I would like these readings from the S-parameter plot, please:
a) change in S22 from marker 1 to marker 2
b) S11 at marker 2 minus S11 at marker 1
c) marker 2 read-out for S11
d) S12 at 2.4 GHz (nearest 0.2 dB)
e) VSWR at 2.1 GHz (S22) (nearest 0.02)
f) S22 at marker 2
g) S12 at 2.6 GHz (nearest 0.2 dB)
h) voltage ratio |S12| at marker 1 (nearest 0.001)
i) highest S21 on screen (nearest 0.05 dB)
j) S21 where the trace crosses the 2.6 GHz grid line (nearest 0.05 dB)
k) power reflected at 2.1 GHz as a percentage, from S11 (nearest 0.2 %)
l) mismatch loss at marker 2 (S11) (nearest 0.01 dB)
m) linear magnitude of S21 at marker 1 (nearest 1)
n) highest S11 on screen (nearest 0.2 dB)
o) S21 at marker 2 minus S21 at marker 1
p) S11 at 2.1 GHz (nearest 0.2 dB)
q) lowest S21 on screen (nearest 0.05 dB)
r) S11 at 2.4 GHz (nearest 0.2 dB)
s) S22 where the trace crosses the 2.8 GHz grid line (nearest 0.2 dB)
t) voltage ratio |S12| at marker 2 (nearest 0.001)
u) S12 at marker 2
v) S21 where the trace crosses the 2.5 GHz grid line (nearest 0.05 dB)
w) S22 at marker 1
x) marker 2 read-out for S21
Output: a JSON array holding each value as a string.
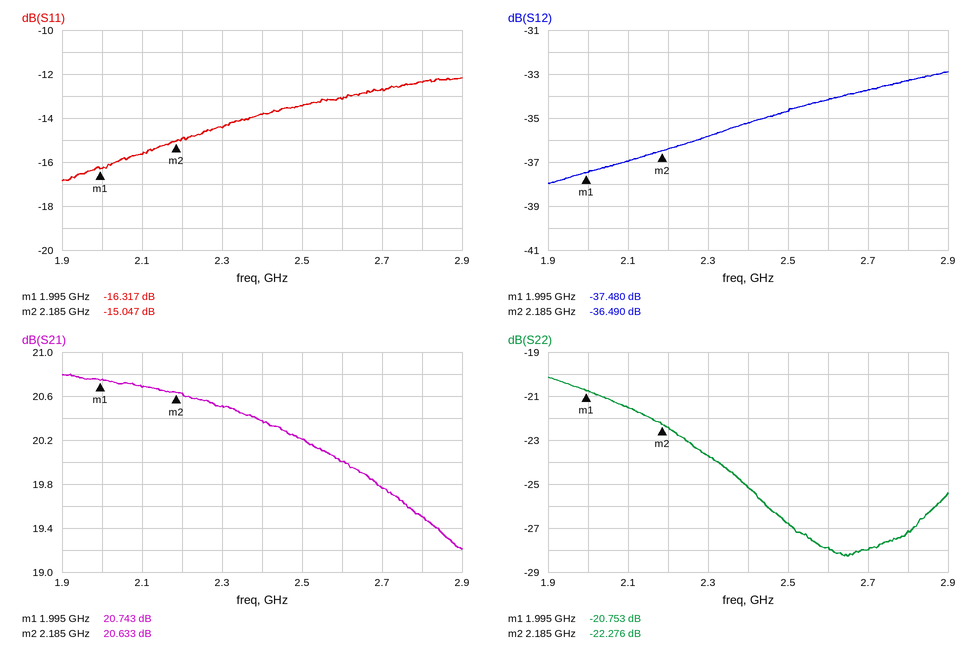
["-1.523 dB", "1.270 dB", "-15.047 dB", "-35.2 dB", "1.18", "-22.276 dB", "-34.2 dB", "0.013", "20.80 dB", "20.00 dB", "2.8 %", "0.14 dB", "11", "-12.2 dB", "-0.110 dB", "-15.6 dB", "19.20 dB", "-13.8 dB", "-27.2 dB", "0.015", "-36.490 dB", "20.20 dB", "-20.753 dB", "20.633 dB"]
